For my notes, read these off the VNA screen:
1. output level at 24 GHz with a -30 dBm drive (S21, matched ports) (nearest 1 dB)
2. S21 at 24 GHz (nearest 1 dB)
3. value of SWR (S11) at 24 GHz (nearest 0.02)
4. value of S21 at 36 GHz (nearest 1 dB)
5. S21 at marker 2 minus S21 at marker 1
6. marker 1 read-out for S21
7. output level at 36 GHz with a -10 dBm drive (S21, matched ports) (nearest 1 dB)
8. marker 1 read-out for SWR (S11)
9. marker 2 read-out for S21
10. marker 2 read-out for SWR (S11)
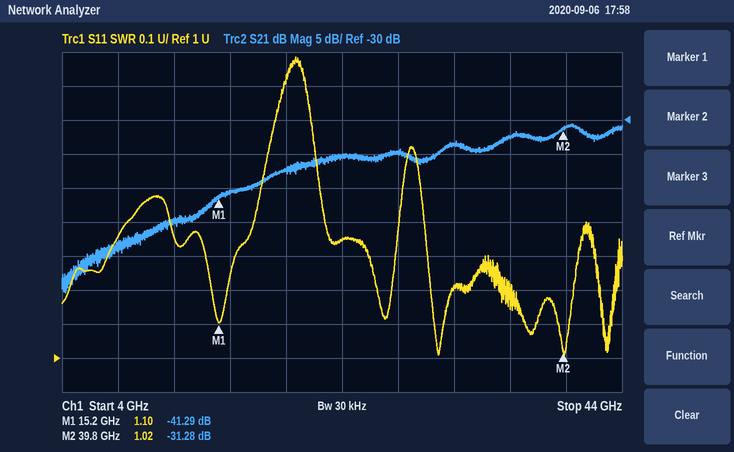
-65 dBm
-35 dB
1.34
-32 dB
10.01 dB
-41.29 dB
-42 dBm
1.10
-31.28 dB
1.02
